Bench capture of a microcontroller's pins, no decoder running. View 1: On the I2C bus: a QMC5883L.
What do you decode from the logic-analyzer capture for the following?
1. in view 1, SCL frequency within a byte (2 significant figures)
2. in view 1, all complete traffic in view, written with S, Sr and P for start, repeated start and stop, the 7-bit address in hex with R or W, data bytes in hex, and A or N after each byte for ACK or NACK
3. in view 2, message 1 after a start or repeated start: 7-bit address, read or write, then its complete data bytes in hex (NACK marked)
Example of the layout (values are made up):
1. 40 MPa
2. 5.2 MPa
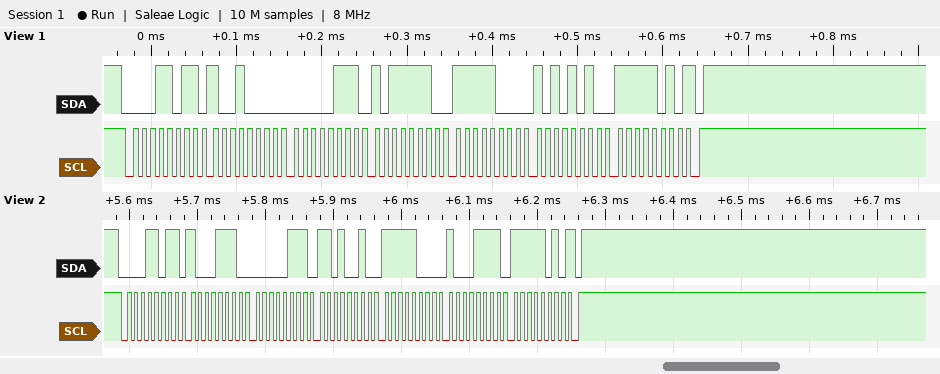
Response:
1. 100 kHz
2. S 0DR A 90 A 07 A BE A F8 A AA A FA N P
3. 0x0D read: 8E 07 D2 F8 8F FA NACK
